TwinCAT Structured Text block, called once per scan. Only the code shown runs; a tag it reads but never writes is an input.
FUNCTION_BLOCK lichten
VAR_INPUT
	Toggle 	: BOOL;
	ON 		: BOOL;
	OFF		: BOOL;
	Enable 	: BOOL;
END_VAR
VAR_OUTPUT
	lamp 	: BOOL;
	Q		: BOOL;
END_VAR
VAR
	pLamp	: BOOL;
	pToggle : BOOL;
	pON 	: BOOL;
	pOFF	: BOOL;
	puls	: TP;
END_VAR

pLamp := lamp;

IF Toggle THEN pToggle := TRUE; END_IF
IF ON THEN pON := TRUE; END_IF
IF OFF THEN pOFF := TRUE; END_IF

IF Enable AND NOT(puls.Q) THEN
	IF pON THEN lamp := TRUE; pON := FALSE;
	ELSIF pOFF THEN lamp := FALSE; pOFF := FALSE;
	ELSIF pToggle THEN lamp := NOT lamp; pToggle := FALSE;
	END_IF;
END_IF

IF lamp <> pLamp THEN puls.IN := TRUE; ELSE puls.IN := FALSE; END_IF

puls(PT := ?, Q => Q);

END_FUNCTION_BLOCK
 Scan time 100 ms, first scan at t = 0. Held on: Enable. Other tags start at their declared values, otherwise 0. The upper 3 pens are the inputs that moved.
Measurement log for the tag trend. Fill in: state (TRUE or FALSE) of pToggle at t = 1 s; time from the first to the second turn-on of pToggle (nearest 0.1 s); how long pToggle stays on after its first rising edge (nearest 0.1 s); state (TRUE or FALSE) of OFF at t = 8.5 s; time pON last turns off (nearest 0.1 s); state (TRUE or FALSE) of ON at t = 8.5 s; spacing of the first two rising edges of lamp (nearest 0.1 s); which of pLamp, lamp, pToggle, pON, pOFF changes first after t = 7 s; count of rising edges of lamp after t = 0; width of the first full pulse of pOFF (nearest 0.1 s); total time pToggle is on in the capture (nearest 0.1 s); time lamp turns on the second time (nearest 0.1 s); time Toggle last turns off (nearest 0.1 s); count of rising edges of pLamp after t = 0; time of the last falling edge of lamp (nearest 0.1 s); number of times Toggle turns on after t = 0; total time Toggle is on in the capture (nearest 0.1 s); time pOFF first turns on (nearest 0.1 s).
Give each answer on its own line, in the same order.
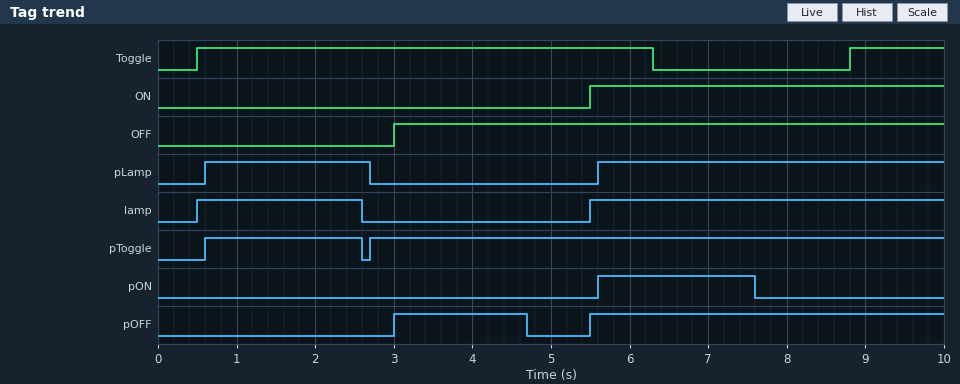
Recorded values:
TRUE
2.1 s
2.0 s
TRUE
7.6 s
TRUE
5.0 s
pON
2
1.7 s
9.3 s
5.5 s
6.3 s
2
2.6 s
2
7.0 s
3.0 s
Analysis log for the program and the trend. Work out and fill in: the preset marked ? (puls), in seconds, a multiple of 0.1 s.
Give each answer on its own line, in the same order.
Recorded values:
2.0 s
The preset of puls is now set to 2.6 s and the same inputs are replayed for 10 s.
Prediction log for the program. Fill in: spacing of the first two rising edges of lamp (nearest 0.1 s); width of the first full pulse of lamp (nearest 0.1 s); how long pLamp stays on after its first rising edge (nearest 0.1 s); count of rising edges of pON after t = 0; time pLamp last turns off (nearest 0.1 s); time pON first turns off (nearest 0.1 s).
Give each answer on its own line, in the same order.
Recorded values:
5.4 s
2.7 s
2.7 s
2
3.3 s
5.9 s
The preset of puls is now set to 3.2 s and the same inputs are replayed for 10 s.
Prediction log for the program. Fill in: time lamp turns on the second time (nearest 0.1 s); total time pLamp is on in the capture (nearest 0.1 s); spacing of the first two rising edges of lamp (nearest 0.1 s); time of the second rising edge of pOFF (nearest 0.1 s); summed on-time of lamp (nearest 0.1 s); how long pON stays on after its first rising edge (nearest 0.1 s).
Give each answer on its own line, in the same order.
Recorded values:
7.1 s
6.1 s
6.6 s
3.9 s
6.2 s
1.6 s
